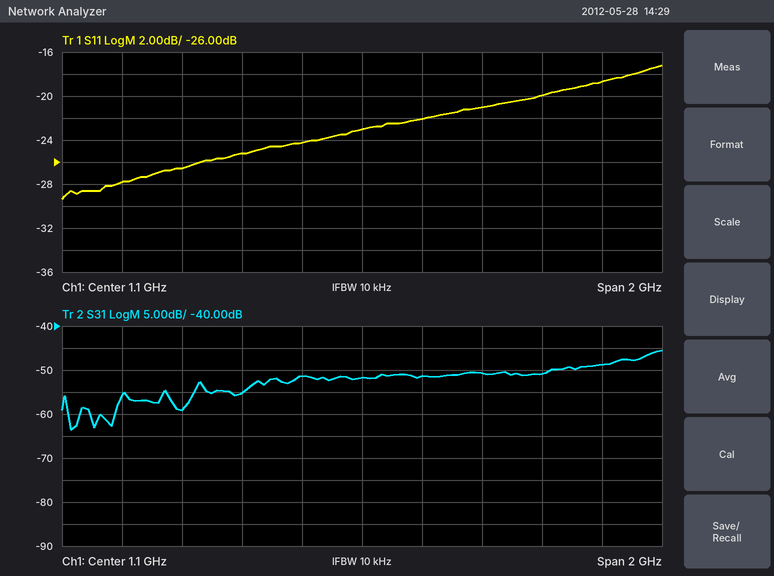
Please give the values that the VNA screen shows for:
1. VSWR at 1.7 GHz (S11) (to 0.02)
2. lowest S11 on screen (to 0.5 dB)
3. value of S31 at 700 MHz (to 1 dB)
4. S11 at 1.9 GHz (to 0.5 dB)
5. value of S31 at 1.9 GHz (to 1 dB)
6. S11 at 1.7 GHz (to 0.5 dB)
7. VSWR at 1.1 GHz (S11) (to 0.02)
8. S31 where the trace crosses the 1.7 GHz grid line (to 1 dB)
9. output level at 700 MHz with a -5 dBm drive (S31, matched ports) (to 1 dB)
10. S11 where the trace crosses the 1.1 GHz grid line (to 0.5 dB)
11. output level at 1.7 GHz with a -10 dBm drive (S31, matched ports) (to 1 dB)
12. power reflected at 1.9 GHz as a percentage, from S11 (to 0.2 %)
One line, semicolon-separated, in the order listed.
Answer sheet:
1.22; -29.5 dB; -55 dB; -18.5 dB; -49 dB; -20.0 dB; 1.16; -51 dB; -60 dBm; -23.0 dB; -61 dBm; 1.4 %
